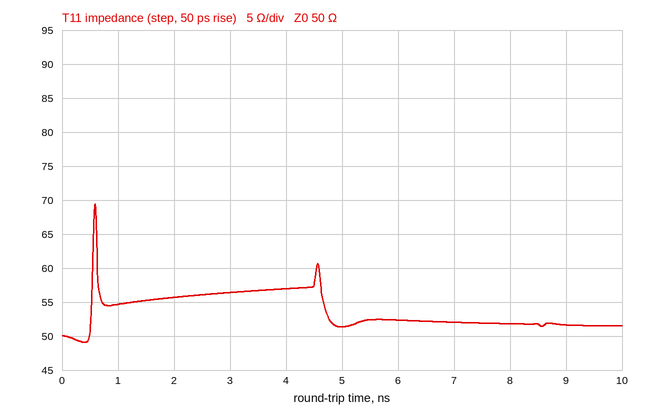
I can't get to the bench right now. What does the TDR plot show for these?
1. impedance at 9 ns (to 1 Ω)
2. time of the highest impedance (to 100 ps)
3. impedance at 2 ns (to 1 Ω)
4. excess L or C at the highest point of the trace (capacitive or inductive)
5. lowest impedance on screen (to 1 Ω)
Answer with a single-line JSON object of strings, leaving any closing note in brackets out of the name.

{"impedance at 9 ns": "52 Ω", "time of the highest impedance": "600 ps", "impedance at 2 ns": "56 Ω", "excess L or C at the highest point of the trace": "inductive", "lowest impedance on screen": "49 Ω"}
